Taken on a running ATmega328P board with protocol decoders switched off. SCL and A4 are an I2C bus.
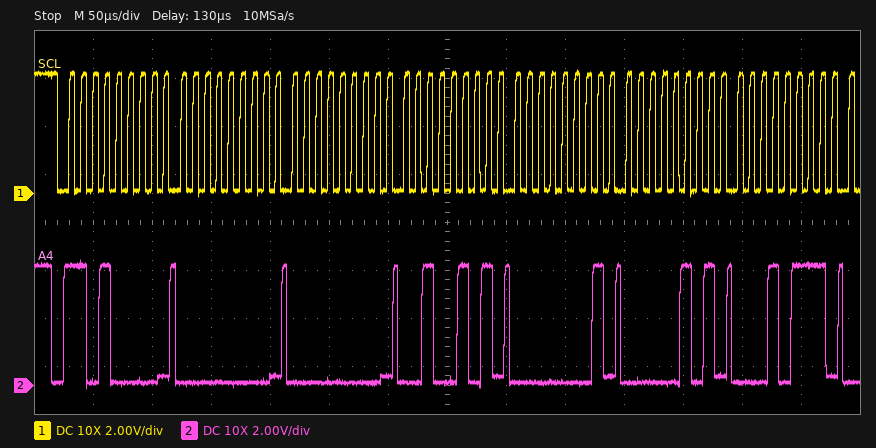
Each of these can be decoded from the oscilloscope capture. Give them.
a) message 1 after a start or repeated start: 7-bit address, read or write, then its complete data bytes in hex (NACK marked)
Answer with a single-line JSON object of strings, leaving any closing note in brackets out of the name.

{"message 1 after a start or repeated start: 7-bit address, read or write, then its complete data bytes in hex": "0x68 write: 00 00 25 01 05 17"}
